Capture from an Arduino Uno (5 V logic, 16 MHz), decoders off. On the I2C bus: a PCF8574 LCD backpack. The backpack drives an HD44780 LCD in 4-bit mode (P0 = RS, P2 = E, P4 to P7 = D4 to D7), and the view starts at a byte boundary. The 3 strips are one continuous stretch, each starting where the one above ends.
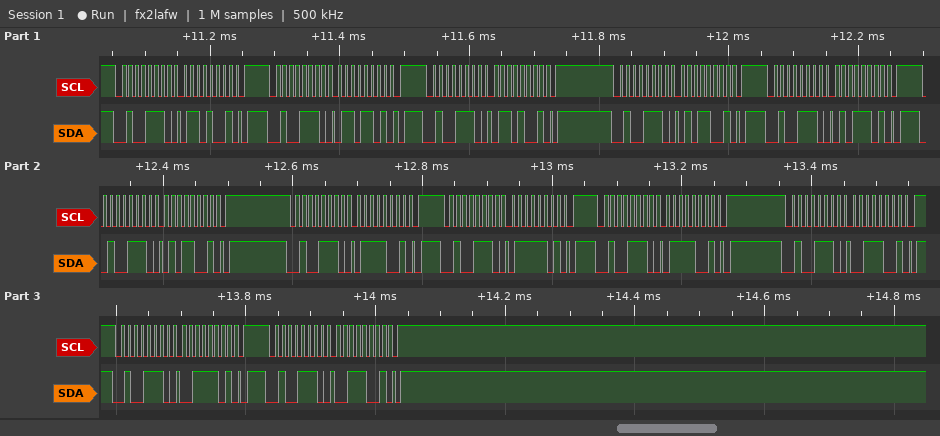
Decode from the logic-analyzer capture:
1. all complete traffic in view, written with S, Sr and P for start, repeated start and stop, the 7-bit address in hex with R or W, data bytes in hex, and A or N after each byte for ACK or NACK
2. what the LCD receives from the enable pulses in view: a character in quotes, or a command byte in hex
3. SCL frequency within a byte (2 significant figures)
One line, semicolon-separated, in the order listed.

S 27W A 69 A P S 27W A 6D A P S 27W A 69 A P S 27W A 59 A P S 27W A 5D A P S 27W A 59 A P S 27W A 79 A P S 27W A 7D A P S 27W A 79 A P S 27W A 39 A P S 27W A 3D A P S 27W A 39 A P; 'e' 's'; 100 kHz
